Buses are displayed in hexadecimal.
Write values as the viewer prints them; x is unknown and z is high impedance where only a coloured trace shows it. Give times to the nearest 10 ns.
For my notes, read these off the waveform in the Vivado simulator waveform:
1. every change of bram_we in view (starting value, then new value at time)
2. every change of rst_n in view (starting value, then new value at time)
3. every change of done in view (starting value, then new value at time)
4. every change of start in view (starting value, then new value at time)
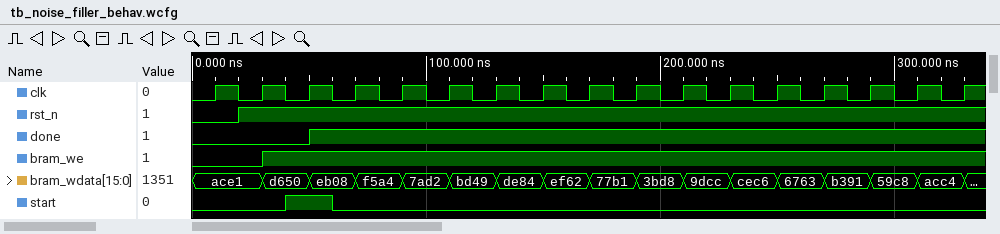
0, 1 at 30 ns
0, 1 at 20 ns
0, 1 at 50 ns
0, 1 at 40 ns, 0 at 60 ns
